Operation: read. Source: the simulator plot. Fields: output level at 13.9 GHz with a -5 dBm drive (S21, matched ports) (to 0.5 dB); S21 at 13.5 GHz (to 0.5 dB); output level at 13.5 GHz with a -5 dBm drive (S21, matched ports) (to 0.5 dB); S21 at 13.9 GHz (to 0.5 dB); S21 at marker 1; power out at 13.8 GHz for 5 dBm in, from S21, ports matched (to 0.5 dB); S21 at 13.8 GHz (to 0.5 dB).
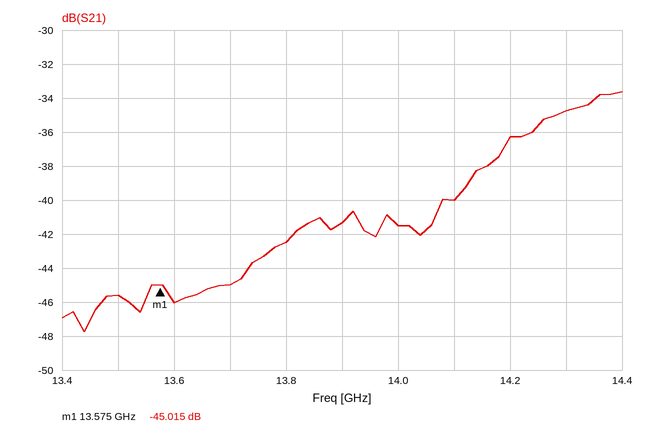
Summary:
-46.5 dBm
-45.5 dB
-50.5 dBm
-41.5 dB
-45.015 dB
-37.5 dBm
-42.5 dB
